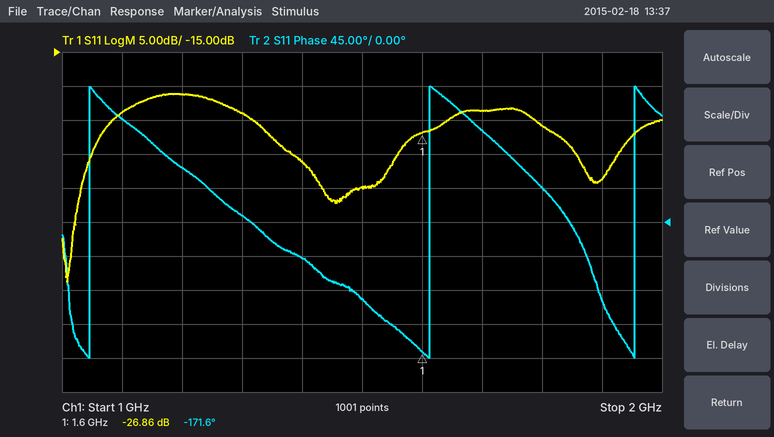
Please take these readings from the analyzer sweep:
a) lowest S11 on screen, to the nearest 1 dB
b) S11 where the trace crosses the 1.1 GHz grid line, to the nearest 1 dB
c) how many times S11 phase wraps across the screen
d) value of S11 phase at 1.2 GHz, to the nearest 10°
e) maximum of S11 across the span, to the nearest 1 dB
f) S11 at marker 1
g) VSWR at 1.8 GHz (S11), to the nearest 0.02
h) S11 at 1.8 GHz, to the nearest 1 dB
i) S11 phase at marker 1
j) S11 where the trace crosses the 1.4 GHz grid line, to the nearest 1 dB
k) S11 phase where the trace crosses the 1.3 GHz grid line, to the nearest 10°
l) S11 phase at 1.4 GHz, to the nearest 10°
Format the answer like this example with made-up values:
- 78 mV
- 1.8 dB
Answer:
- -49 dB
- -24 dB
- 3
- 70°
- -21 dB
- -26.86 dB
- 1.10
- -26 dB
- -171.6°
- -31 dB
- 10°
- -50°
